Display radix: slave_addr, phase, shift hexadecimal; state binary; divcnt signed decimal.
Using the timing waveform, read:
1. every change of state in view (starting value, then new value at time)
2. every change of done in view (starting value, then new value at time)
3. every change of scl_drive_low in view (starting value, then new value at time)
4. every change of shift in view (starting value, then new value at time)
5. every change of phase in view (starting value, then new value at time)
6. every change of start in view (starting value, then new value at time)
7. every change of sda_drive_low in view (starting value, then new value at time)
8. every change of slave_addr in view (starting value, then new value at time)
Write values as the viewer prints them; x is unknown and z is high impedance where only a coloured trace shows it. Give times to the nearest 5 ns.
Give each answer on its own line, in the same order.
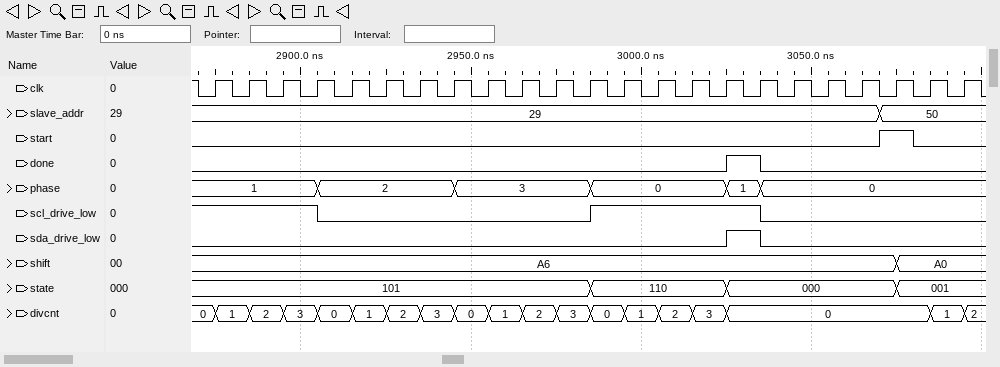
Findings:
101, 110 at 2985 ns, 000 at 3025 ns, 001 at 3075 ns
0, 1 at 3025 ns, 0 at 3035 ns
1, 0 at 2905 ns, 1 at 2985 ns, 0 at 3035 ns
A6, A0 at 3075 ns
1, 2 at 2905 ns, 3 at 2945 ns, 0 at 2985 ns, 1 at 3025 ns, 0 at 3035 ns
0, 1 at 3070 ns, 0 at 3080 ns
0, 1 at 3025 ns, 0 at 3035 ns
29, 50 at 3070 ns
